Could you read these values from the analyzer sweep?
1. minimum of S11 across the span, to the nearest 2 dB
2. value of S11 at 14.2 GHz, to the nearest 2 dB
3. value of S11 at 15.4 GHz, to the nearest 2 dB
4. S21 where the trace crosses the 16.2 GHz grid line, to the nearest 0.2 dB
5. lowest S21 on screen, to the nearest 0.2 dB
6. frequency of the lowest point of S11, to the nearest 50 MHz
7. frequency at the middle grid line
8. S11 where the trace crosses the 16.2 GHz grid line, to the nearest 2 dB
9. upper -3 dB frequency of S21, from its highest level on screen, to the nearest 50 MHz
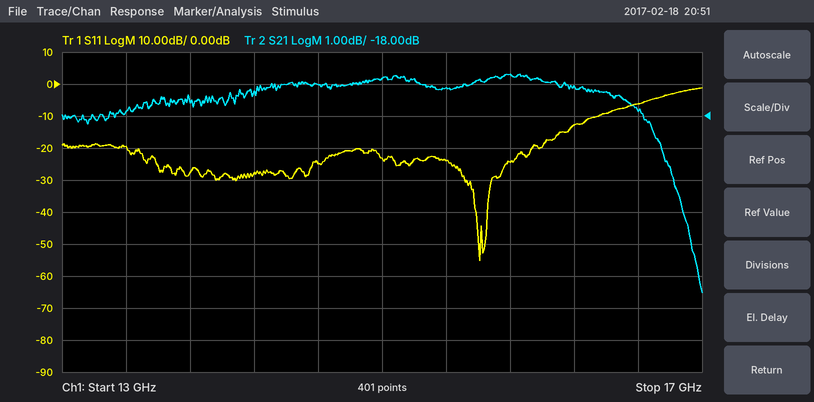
-56 dB
-28 dB
-24 dB
-17.0 dB
-23.6 dB
15.60 GHz
15 GHz
-12 dB
16.80 GHz
